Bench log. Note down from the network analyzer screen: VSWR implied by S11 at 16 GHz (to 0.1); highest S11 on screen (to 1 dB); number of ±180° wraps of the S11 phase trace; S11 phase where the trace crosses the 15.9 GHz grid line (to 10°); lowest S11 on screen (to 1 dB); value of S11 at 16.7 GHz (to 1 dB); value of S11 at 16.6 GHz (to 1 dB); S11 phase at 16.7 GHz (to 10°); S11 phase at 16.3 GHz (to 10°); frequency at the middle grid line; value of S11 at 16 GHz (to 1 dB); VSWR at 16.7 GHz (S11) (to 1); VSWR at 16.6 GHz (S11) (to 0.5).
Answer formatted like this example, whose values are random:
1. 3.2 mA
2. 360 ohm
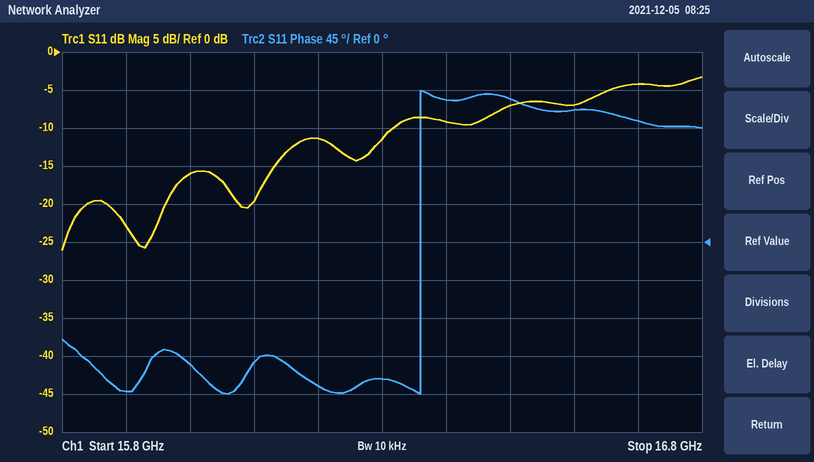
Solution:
1. 1.4
2. -3 dB
3. 1
4. -180°
5. -26 dB
6. -4 dB
7. -7 dB
8. 140°
9. -160°
10. 16.3 GHz
11. -16 dB
12. 4
13. 2.5
